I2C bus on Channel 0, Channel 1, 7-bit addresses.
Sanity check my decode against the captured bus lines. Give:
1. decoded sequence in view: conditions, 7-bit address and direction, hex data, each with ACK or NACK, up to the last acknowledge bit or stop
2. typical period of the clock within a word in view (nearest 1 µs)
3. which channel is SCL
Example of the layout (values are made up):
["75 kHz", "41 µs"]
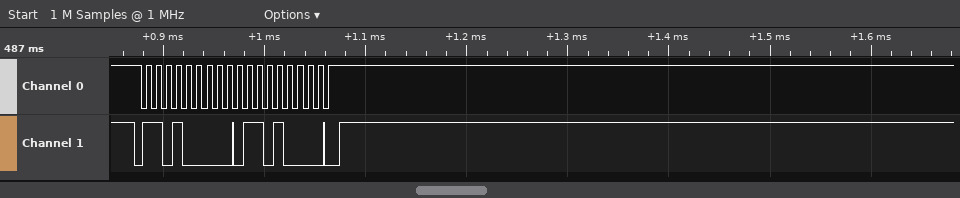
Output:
["start, address 68 write ACK, 68 ACK, stop", "10 µs", "Channel 0"]
